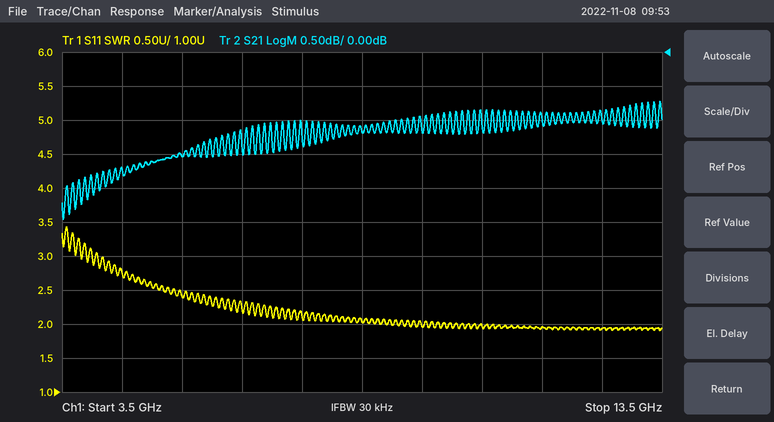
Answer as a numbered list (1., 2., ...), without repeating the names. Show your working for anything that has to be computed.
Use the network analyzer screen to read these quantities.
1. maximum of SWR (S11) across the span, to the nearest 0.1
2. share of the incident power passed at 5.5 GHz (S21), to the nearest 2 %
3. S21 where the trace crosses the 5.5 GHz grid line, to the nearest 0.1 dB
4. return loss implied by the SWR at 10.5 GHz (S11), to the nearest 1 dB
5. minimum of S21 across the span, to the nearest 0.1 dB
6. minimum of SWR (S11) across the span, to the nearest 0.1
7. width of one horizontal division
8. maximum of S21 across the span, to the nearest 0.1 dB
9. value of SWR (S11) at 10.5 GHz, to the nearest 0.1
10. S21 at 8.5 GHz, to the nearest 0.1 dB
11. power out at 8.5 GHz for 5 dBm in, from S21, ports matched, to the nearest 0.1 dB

1. 3.4
2. 10^(-1.5/10) ≈ 70.8 %, so 70 % to the nearest 2 %
3. -1.5 dB
4. −20 log10((2 − 1)/(2 + 1)) ≈ 10 dB
5. -2.5 dB
6. 1.9
7. 1 GHz
8. -0.7 dB
9. 2.0
10. -1.2 dB
11. 5 dBm + (-1.2 dB) = 3.8 dBm
